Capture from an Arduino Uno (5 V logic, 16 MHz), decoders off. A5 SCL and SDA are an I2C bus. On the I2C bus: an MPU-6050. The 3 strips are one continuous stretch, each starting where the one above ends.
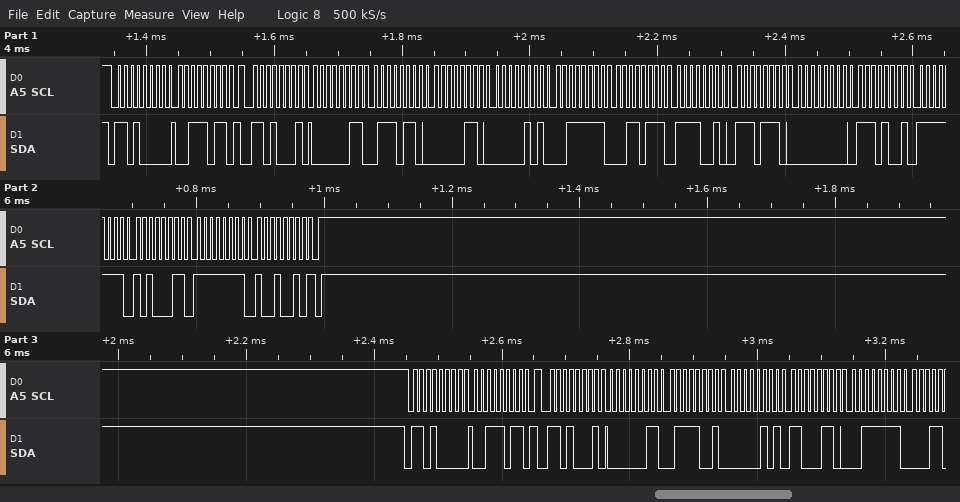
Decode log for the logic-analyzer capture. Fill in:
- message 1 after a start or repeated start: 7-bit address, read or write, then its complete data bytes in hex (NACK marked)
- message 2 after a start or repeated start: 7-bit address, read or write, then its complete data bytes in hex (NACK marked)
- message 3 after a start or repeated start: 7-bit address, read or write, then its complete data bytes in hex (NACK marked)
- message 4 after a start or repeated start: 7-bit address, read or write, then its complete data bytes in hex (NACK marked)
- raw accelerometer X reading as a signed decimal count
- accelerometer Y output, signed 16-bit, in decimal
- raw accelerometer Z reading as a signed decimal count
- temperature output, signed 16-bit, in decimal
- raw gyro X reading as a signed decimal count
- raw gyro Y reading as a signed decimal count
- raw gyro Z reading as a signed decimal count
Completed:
0x68 write: 3B
0x68 read: 03 76 06 05 3F 37 F2 EE 00 E9 FF A3 FF 92 NACK
0x68 write: 3B
0x68 read: 03 79 05 C6 3F
886
1541
16183
-3346
233
-93
-110
